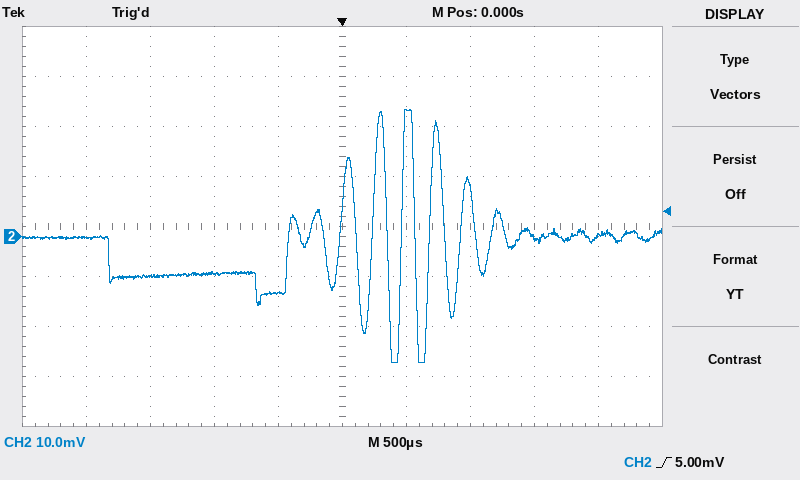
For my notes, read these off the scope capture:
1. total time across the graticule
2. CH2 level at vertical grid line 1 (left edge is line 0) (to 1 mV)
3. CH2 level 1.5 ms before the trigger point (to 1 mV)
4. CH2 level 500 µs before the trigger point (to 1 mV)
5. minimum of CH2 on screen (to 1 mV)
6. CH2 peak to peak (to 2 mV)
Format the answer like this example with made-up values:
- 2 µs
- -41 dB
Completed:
- 5 ms
- 0 mV
- -8 mV
- -11 mV
- -25 mV
- 50 mV
